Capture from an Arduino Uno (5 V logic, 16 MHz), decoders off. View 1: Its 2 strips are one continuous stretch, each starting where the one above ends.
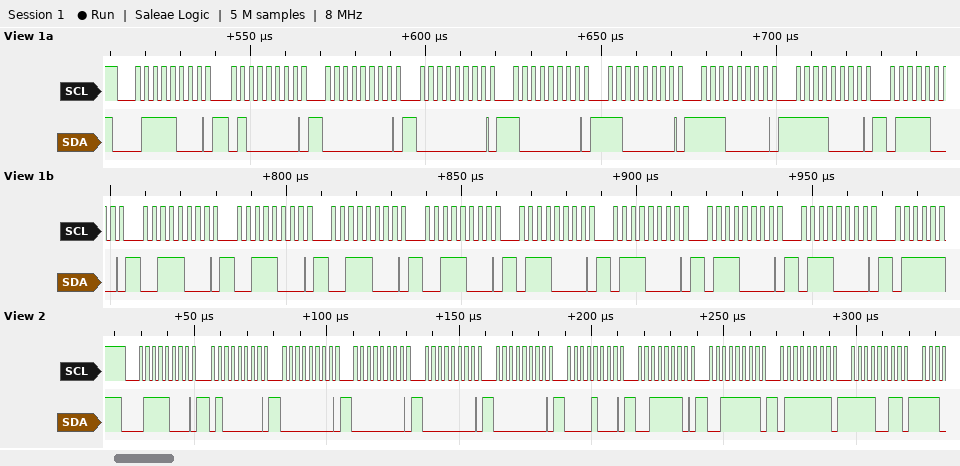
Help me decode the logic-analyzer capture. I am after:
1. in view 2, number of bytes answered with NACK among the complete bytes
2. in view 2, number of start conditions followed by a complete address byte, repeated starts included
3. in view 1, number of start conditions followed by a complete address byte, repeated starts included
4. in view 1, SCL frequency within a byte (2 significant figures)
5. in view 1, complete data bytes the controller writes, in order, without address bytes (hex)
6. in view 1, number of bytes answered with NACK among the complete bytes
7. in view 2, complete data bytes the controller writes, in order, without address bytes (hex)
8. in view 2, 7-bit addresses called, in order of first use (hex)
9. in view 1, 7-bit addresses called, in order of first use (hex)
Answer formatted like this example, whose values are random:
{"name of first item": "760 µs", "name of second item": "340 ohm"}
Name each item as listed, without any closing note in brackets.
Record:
{"in view 2, number of bytes answered with NACK among the complete bytes": "0", "in view 2, number of start conditions followed by a complete address byte, repeated starts included": "1", "in view 1, number of start conditions followed by a complete address byte, repeated starts included": "1", "in view 1, SCL frequency within a byte": "400 kHz", "in view 1, complete data bytes the controller writes, in order, without address bytes": "40 00 00 80 C0 E0 F0 78 38 38 38 38 70 70 70 70", "in view 1, number of bytes answered with NACK among the complete bytes": "0", "in view 2, complete data bytes the controller writes, in order, without address bytes": "40 00 00 00 00 08 3E 3F 7F F3", "in view 2, 7-bit addresses called, in order of first use": "0x3C", "in view 1, 7-bit addresses called, in order of first use": "0x3C"}
